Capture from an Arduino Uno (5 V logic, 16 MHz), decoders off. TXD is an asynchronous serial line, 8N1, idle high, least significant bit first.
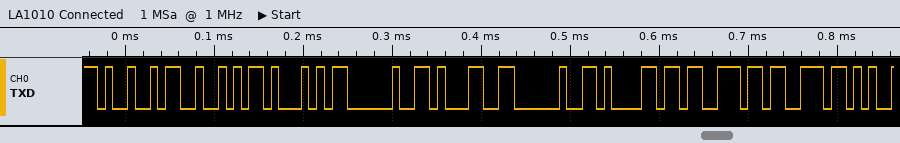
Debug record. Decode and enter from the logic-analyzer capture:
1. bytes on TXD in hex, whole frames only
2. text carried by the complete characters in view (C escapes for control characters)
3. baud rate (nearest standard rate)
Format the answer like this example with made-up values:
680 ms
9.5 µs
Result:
0x49 0x52 0x51 0x20 0x31 0x20 0x61 0x73 0x73
"IRQ 1 ass"
115200 baud
